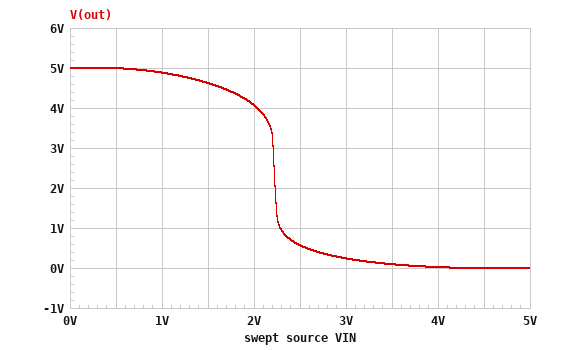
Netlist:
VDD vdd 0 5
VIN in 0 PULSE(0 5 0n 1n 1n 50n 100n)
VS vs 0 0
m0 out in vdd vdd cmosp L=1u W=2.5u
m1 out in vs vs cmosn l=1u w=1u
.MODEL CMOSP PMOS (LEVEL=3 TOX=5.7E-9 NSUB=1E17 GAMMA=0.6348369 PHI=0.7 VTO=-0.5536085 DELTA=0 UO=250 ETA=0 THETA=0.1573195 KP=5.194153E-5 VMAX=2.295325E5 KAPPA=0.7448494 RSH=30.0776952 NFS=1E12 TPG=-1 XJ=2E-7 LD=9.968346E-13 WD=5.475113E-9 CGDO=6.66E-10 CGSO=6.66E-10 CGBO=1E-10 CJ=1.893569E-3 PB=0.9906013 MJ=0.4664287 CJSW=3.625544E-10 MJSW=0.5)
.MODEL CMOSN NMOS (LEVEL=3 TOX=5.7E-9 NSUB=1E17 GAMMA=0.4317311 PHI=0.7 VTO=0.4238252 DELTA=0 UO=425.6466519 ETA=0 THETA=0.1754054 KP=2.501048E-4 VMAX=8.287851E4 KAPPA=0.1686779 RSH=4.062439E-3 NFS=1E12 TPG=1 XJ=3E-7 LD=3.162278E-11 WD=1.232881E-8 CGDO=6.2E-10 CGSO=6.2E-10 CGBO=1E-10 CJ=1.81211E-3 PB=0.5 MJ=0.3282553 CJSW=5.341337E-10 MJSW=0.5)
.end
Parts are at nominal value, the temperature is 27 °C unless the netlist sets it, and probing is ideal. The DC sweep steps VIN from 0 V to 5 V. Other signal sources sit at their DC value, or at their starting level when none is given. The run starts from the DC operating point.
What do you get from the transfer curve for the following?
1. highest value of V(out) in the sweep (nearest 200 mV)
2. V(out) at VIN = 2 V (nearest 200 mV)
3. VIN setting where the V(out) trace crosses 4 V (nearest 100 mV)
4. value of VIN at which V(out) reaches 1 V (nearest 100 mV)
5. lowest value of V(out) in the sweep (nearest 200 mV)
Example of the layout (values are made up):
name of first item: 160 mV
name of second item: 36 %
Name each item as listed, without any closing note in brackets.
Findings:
highest value of V(out) in the sweep: 5.0 V
V(out) at VIN = 2 V: 4.0 V
VIN setting where the V(out) trace crosses 4 V: 2.0 V
value of VIN at which V(out) reaches 1 V: 2.3 V
lowest value of V(out) in the sweep: 0 V
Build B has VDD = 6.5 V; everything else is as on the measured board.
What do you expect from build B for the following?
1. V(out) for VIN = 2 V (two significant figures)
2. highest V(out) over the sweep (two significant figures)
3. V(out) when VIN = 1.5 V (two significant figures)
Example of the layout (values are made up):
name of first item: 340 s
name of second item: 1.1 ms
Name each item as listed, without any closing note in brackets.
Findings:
V(out) for VIN = 2 V: 5.9 V
highest V(out) over the sweep: 6.5 V
V(out) when VIN = 1.5 V: 6.2 V
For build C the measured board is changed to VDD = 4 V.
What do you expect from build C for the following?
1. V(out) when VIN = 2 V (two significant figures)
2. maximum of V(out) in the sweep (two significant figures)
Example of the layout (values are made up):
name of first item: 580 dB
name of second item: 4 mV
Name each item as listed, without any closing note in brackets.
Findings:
V(out) when VIN = 2 V: 400 mV
maximum of V(out) in the sweep: 4.0 V
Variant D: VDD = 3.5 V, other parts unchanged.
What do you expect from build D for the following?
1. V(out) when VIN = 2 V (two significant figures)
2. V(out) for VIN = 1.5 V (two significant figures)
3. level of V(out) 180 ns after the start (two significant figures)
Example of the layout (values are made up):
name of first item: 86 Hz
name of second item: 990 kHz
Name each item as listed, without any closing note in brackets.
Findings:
V(out) when VIN = 2 V: 160 mV
V(out) for VIN = 1.5 V: 2.6 V
level of V(out) 180 ns after the start: 3.5 V
